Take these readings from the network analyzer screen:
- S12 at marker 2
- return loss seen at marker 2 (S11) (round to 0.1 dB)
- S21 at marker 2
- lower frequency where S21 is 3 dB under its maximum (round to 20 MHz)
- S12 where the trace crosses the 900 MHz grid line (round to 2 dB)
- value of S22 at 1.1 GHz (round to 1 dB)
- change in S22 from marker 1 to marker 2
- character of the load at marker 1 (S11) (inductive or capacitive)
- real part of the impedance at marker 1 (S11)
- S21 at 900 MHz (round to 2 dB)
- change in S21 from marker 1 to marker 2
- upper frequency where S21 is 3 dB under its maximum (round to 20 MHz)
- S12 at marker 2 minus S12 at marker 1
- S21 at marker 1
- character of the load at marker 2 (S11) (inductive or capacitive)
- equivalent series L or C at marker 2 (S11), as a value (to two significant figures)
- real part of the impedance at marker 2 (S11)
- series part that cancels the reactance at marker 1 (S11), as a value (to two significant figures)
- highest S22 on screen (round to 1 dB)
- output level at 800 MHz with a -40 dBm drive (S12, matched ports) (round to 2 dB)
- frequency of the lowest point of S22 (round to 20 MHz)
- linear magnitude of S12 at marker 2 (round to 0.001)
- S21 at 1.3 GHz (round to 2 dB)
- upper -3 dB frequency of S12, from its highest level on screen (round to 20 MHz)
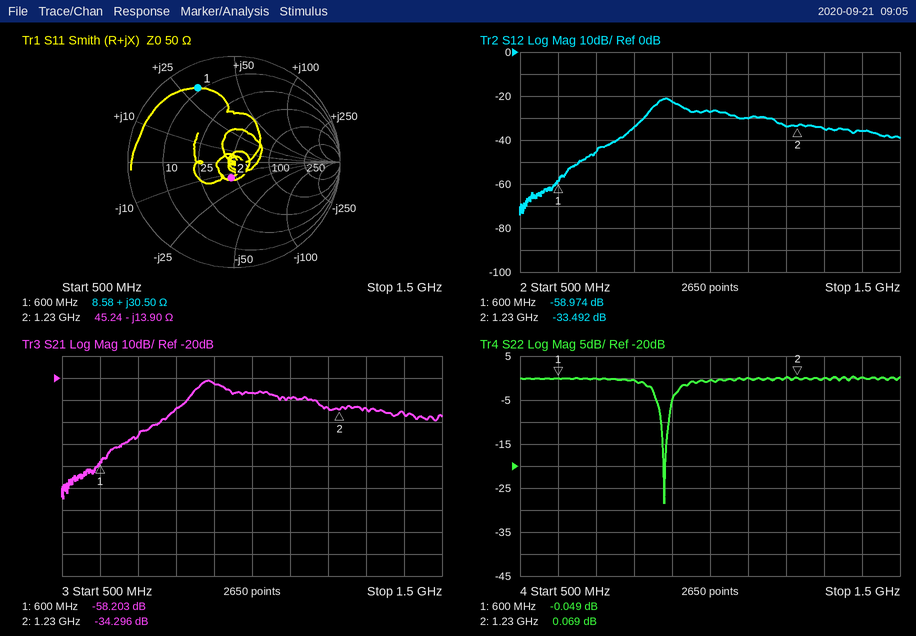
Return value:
-33.492 dB
16.3 dB
-34.296 dB
860 MHz
-22 dB
0 dB
0.118 dB
inductive
8.58 Ω
-22 dB
23.907 dB
920 MHz
25.482 dB
-58.203 dB
capacitive
9.3 pF
45.24 Ω
8.7 pF
0 dB
-74 dBm
880 MHz
0.021
-34 dB
920 MHz
